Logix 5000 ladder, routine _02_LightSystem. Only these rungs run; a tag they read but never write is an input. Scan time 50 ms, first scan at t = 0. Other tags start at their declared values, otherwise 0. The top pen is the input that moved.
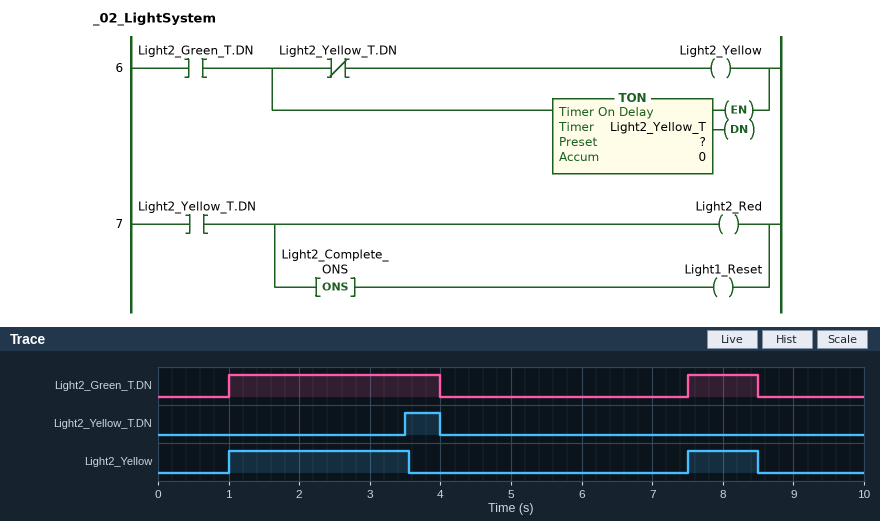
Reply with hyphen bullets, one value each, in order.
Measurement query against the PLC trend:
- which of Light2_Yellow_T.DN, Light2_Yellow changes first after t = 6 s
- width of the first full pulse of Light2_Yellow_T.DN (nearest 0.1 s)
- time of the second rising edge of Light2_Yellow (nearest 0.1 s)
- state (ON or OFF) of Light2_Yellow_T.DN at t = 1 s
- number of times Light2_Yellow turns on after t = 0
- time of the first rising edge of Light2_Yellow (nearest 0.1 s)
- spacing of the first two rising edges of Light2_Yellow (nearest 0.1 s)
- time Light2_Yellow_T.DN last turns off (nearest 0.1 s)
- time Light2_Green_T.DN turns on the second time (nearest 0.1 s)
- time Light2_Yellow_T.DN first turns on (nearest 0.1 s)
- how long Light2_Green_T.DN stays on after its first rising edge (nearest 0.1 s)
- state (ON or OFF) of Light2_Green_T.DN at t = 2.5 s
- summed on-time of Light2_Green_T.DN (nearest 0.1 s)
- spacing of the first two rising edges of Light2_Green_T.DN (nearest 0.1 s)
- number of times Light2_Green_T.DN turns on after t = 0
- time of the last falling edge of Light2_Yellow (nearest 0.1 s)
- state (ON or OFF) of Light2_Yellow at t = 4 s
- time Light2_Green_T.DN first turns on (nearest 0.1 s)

- Light2_Yellow
- 0.5 s
- 7.5 s
- OFF
- 2
- 1.0 s
- 6.5 s
- 4.0 s
- 7.5 s
- 3.5 s
- 3.0 s
- ON
- 4.0 s
- 6.5 s
- 2
- 8.5 s
- OFF
- 1.0 s
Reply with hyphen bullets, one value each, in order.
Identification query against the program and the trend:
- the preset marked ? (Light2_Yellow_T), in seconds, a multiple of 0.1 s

- 2.5 s
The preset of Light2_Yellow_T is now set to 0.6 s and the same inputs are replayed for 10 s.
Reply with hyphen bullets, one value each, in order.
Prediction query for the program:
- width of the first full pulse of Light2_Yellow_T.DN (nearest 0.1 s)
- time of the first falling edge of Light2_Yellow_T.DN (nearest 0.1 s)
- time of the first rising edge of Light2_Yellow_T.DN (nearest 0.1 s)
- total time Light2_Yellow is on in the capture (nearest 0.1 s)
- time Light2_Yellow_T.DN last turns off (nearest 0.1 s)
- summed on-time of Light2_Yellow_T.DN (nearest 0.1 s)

- 2.4 s
- 4.0 s
- 1.6 s
- 1.3 s
- 8.5 s
- 2.8 s
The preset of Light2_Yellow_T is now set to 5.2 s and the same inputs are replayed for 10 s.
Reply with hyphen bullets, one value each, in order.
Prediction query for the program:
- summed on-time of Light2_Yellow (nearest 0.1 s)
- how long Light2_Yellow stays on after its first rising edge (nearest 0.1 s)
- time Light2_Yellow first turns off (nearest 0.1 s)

- 4.0 s
- 3.0 s
- 4.0 s
